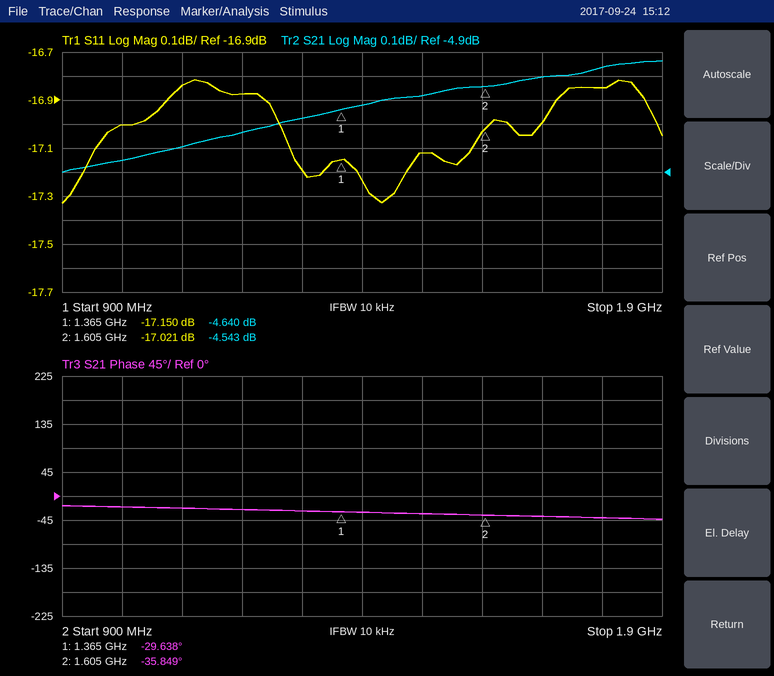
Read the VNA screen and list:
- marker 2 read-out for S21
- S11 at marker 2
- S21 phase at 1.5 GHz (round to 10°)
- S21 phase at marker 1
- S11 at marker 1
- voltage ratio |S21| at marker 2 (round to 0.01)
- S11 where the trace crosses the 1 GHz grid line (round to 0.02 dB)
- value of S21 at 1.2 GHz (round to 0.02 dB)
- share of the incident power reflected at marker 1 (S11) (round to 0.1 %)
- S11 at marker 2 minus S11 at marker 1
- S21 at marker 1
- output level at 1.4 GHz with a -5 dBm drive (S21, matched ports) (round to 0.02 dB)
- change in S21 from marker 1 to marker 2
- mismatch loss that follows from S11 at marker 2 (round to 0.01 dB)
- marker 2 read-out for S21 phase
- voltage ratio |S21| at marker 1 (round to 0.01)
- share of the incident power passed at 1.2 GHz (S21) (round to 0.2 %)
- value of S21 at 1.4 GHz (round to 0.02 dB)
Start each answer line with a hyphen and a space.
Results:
- -4.543 dB
- -17.021 dB
- -30°
- -29.638°
- -17.150 dB
- 0.59
- -17.00 dB
- -4.74 dB
- 1.9 %
- 0.129 dB
- -4.640 dB
- -9.62 dBm
- 0.097 dB
- 0.09 dB
- -35.849°
- 0.59
- 33.6 %
- -4.62 dB
